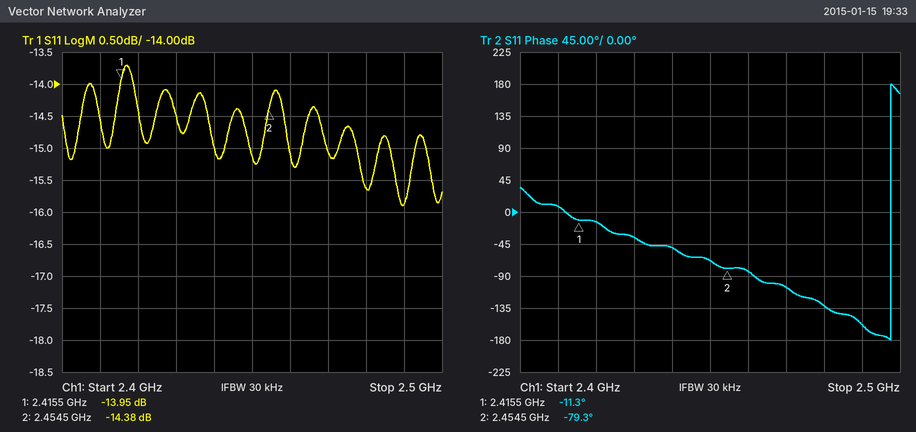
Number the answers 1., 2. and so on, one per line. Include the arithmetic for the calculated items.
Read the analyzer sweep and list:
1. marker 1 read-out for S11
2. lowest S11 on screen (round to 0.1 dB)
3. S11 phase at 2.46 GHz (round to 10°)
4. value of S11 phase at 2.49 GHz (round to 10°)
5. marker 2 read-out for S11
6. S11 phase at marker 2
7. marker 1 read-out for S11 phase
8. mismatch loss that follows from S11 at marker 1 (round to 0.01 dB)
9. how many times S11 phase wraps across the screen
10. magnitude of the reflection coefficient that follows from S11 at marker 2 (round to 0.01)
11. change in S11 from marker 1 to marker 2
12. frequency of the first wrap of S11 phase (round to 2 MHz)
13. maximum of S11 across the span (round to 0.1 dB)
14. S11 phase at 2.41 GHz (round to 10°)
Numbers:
1. -13.95 dB
2. -15.9 dB
3. -80°
4. -160°
5. -14.38 dB
6. -79.3°
7. -11.3°
8. −10 log10(1 − 10^(-13.95/10)) ≈ 0.18 dB
9. 1
10. 10^(-14.38/20) ≈ 0.19
11. -14.38 − (-13.95) = -0.43 dB
12. 2.498 GHz
13. -13.7 dB
14. 10°
